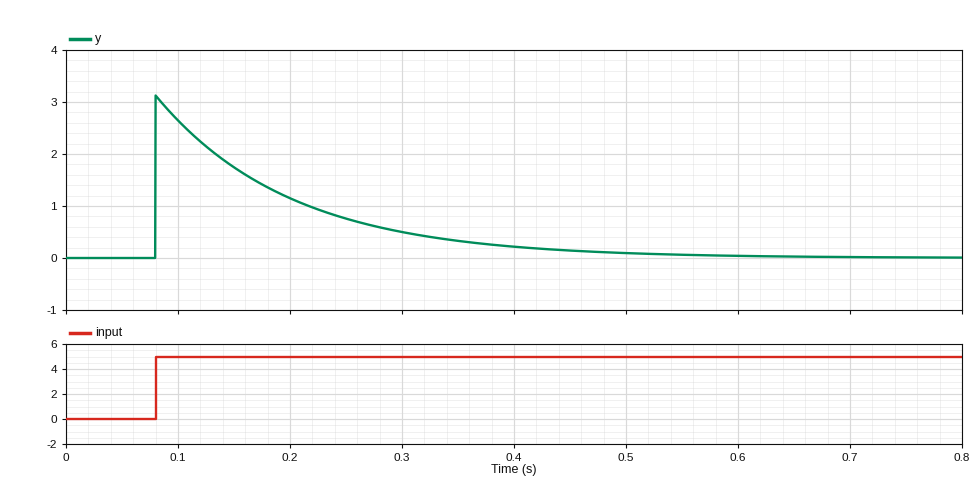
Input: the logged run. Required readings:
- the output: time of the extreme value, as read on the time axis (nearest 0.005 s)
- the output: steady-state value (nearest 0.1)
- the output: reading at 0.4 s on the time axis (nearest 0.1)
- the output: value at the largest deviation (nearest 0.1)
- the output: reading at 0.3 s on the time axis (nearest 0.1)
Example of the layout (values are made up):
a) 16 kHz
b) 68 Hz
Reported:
a) 0.080 s
b) 0.0
c) 0.2
d) 3.1
e) 0.5
